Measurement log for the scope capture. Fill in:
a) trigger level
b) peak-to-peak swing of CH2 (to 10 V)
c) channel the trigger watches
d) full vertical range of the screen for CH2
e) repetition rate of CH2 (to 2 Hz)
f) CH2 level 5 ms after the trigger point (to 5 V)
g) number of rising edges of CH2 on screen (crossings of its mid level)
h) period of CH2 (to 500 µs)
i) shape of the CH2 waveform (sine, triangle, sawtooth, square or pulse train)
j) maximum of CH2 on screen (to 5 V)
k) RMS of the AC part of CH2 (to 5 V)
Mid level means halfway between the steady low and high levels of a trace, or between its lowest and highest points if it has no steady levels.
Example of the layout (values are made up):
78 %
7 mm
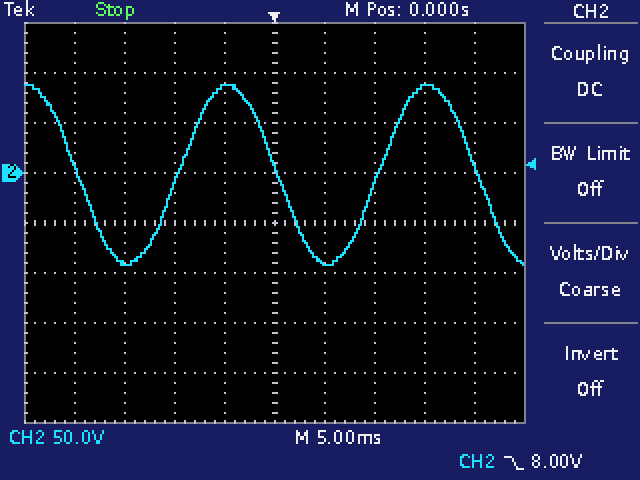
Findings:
8.00 V
180 V
CH2
400 V
50 Hz
-90 V
2
20.0 ms
sine
90 V
65 V
